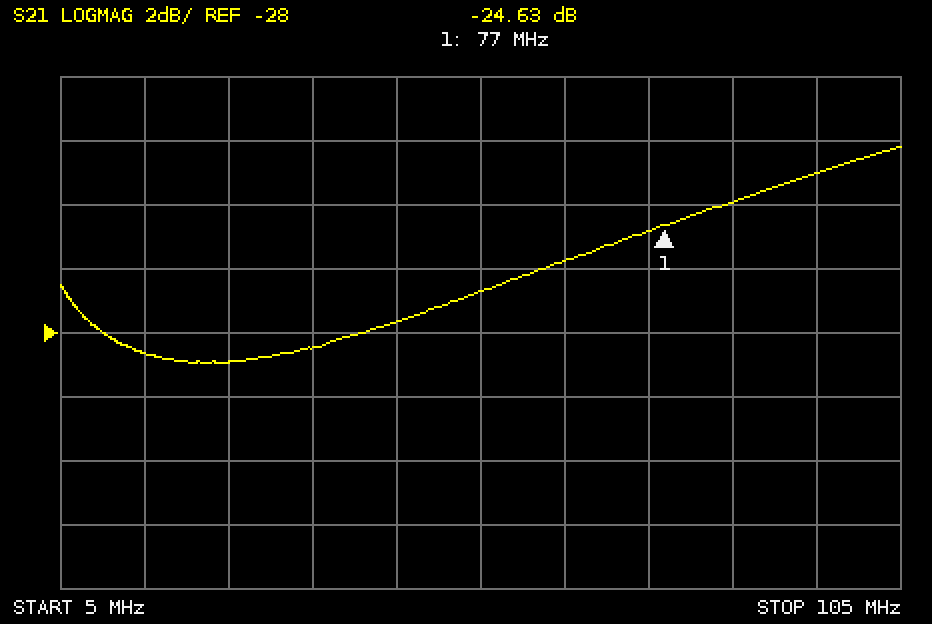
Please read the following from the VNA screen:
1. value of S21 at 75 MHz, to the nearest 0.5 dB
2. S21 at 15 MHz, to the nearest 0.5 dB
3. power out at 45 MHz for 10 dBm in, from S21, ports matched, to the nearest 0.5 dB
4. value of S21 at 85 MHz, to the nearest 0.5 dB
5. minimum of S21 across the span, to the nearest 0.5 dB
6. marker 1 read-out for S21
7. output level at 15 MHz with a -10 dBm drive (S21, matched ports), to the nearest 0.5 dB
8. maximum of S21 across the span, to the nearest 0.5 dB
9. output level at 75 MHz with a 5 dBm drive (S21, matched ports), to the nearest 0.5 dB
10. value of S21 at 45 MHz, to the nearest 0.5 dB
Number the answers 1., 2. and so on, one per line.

1. -25.0 dB
2. -28.5 dB
3. -17.5 dBm
4. -24.0 dB
5. -29.0 dB
6. -24.63 dB
7. -38.5 dBm
8. -22.0 dB
9. -20.0 dBm
10. -27.5 dB
